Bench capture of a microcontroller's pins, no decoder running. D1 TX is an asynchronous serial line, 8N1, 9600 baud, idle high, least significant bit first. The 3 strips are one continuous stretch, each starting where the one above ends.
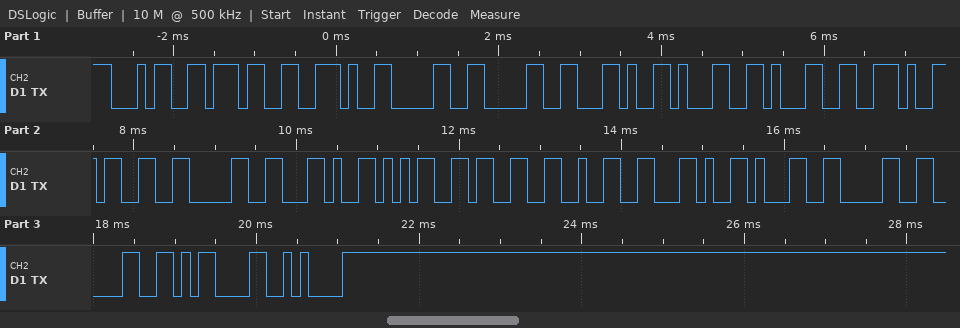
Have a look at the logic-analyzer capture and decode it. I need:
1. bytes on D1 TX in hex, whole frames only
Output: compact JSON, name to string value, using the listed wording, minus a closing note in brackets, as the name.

{"bytes on D1 TX in hex, whole frames only": "34 37 2E 30 30 2C 31 31 2E 33 30 2C 35 33 32 2C 31 30 30 0D 0A"}
